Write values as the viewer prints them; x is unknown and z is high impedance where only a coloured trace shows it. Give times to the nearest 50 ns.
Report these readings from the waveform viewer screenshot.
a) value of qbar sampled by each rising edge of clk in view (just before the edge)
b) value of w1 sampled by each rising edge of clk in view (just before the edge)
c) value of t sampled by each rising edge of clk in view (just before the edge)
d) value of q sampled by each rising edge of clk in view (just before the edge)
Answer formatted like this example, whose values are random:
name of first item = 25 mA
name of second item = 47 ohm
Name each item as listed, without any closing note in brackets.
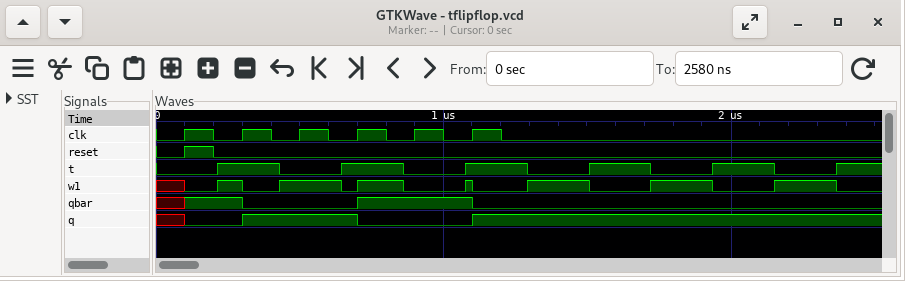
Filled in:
value of qbar sampled by each rising edge of clk in view = x 1 0 0 1 1
value of w1 sampled by each rising edge of clk in view = x 1 1 0 0 1
value of t sampled by each rising edge of clk in view = 0 1 0 1 0 1
value of q sampled by each rising edge of clk in view = x 0 1 1 0 0
